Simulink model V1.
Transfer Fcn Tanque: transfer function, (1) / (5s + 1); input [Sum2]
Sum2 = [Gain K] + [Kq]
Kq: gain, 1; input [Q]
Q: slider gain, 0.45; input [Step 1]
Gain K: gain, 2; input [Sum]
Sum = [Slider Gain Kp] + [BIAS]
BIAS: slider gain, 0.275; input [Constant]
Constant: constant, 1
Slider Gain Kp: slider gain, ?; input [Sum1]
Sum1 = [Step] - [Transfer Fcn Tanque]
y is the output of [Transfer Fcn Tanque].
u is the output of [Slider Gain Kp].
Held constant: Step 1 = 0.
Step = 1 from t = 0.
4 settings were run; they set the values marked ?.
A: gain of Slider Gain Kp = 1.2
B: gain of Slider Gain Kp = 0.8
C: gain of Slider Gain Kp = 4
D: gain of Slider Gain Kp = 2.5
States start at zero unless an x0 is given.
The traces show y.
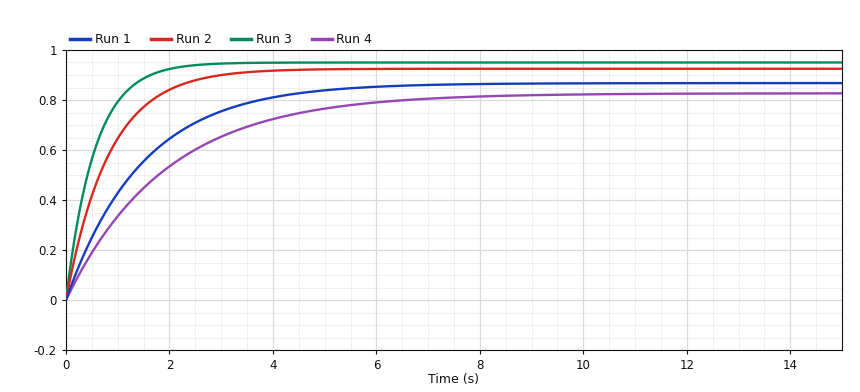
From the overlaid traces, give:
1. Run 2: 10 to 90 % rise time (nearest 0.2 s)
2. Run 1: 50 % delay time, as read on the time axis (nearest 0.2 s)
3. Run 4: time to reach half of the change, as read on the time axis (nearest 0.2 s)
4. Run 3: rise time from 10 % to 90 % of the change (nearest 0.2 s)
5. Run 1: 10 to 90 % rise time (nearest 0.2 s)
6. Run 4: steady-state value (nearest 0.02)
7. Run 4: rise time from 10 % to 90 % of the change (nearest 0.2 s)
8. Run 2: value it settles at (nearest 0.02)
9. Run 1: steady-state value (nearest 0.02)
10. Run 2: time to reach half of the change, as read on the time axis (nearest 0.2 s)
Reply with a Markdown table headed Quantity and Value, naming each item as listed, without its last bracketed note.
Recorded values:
| Quantity | Value |
|---|---|
| Run 2: 10 to 90 % rise time | 1.8 s |
| Run 1: 50 % delay time, as read on the time axis | 1.0 s |
| Run 4: time to reach half of the change, as read on the time axis | 1.4 s |
| Run 3: rise time from 10 % to 90 % of the change | 1.2 s |
| Run 1: 10 to 90 % rise time | 3.2 s |
| Run 4: steady-state value | 0.82 |
| Run 4: rise time from 10 % to 90 % of the change | 4.2 s |
| Run 2: value it settles at | 0.92 |
| Run 1: steady-state value | 0.86 |
| Run 2: time to reach half of the change, as read on the time axis | 0.6 s |
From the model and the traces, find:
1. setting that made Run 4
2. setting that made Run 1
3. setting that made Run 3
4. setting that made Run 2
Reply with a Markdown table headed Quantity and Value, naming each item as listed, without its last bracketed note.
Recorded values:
| Quantity | Value |
|---|---|
| setting that made Run 4 | B |
| setting that made Run 1 | A |
| setting that made Run 3 | C |
| setting that made Run 2 | D |
